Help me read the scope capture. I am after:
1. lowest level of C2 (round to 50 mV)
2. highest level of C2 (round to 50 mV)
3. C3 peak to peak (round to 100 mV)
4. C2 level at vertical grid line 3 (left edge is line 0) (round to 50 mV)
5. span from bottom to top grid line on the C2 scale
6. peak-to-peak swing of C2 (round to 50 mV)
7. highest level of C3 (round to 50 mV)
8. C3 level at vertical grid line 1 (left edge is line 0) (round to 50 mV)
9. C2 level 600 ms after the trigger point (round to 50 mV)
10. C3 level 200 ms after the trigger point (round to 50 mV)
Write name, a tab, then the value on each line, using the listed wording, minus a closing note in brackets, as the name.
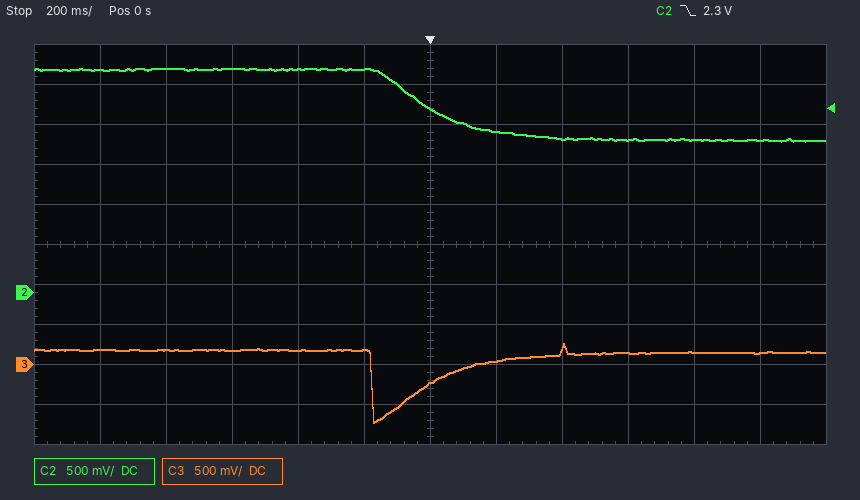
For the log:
lowest level of C2	1.90 V
highest level of C2	2.80 V
C3 peak to peak	1.00 V
C2 level at vertical grid line 3 (left edge is line 0)	2.80 V
span from bottom to top grid line on the C2 scale	5 V
peak-to-peak swing of C2	900 mV
highest level of C3	250 mV
C3 level at vertical grid line 1 (left edge is line 0)	200 mV
C2 level 600 ms after the trigger point	1.90 V
C3 level 200 ms after the trigger point	50 mV
